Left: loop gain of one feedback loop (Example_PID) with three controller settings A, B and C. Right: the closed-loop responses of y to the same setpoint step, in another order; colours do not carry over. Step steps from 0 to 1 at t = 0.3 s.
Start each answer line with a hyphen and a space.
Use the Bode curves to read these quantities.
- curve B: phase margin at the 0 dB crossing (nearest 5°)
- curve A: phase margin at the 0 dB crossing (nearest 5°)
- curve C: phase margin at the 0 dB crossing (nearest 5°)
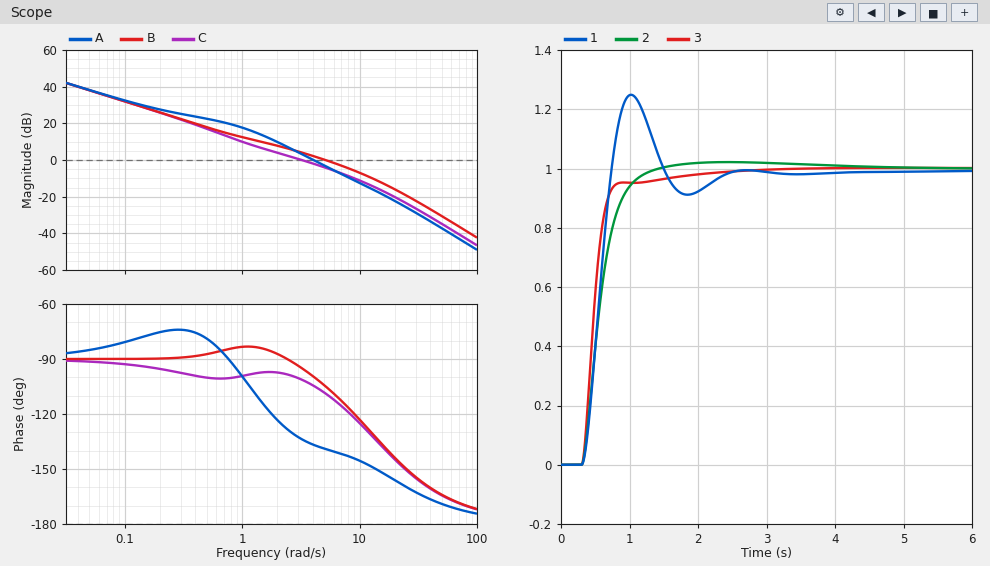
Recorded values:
- 75°
- 45°
- 80°
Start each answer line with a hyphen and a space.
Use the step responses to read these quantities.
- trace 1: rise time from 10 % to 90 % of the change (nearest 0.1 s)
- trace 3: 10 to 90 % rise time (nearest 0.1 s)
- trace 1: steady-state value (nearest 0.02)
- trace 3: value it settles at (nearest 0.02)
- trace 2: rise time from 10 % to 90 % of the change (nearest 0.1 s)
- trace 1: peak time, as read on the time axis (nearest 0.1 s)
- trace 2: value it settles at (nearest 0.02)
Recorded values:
- 0.3 s
- 0.3 s
- 1.00
- 1.00
- 0.5 s
- 1.0 s
- 1.00
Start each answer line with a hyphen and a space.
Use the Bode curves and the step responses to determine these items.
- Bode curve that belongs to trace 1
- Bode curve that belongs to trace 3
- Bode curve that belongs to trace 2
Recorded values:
- A
- B
- C
